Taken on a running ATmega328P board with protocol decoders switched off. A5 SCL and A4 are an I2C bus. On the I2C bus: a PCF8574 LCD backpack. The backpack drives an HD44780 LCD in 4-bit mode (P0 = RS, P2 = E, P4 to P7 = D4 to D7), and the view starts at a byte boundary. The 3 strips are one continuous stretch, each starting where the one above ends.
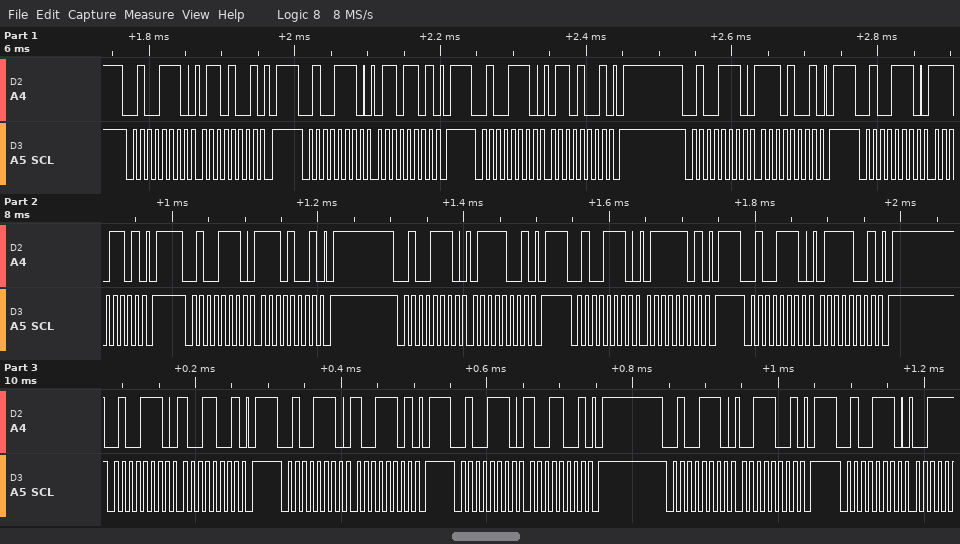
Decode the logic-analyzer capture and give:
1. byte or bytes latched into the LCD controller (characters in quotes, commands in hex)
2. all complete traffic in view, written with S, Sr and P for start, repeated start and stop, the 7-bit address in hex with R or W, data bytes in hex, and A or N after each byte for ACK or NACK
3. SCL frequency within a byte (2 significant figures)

'n' 'y'
S 27W A 69 A P S 27W A 6D A P S 27W A 69 A P S 27W A E9 A P S 27W A ED A P S 27W A E9 A P S 27W A 79 A P S 27W A 7D A P S 27W A 79 A P S 27W A 99 A P S 27W A 9D A P S 27W A 99 A P S 27W A 39 A P S 27W A
100 kHz
